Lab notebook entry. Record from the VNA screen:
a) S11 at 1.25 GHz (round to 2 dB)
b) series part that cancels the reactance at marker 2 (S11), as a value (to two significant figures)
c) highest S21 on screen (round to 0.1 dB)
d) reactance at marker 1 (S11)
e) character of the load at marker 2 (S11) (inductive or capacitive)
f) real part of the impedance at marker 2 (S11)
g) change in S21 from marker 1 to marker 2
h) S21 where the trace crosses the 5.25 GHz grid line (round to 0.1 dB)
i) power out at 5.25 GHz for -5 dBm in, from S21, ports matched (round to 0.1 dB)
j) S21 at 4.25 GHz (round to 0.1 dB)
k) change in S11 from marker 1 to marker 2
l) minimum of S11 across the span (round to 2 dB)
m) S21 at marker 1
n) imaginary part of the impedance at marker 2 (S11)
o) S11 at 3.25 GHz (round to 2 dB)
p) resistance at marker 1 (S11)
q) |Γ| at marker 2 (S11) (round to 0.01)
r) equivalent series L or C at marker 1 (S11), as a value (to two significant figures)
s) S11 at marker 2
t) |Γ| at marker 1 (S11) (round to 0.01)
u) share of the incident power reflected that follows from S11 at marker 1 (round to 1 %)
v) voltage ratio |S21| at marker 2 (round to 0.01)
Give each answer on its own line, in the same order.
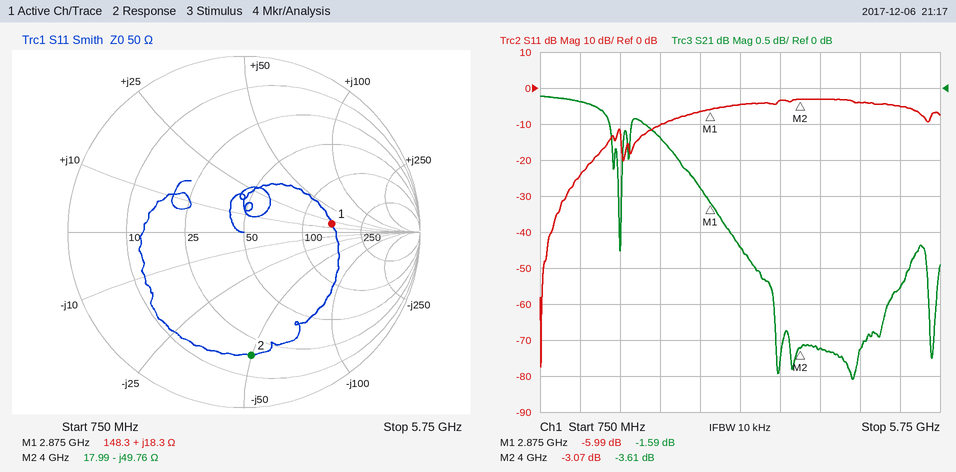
-24 dB
2.0 nH
-0.1 dB
+18.3 Ω
capacitive
17.99 Ω
-2.02 dB
-2.8 dB
-7.8 dBm
-3.6 dB
2.92 dB
-78 dB
-1.59 dB
-49.76 Ω
-4 dB
148.3 Ω
0.70
1.0 nH
-3.07 dB
0.50
25 %
0.66
